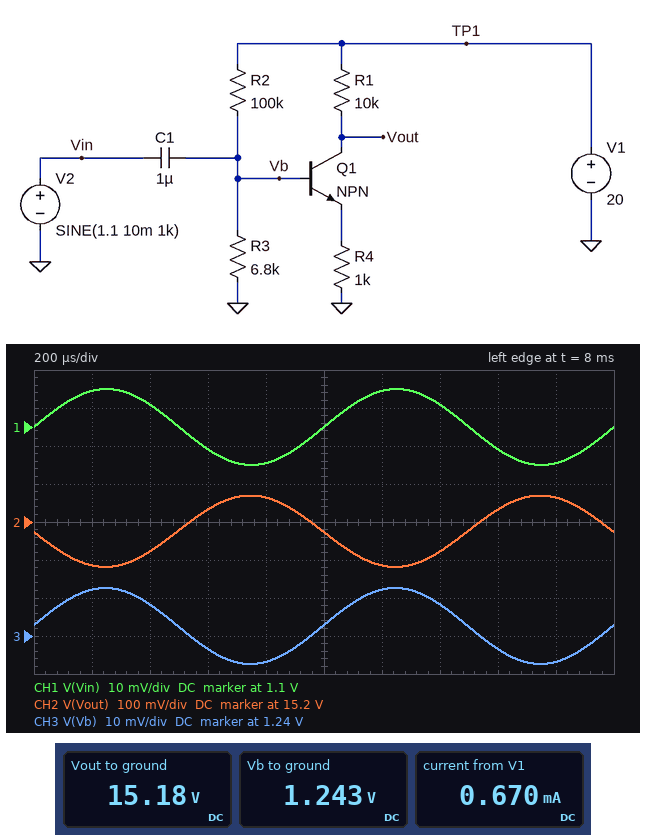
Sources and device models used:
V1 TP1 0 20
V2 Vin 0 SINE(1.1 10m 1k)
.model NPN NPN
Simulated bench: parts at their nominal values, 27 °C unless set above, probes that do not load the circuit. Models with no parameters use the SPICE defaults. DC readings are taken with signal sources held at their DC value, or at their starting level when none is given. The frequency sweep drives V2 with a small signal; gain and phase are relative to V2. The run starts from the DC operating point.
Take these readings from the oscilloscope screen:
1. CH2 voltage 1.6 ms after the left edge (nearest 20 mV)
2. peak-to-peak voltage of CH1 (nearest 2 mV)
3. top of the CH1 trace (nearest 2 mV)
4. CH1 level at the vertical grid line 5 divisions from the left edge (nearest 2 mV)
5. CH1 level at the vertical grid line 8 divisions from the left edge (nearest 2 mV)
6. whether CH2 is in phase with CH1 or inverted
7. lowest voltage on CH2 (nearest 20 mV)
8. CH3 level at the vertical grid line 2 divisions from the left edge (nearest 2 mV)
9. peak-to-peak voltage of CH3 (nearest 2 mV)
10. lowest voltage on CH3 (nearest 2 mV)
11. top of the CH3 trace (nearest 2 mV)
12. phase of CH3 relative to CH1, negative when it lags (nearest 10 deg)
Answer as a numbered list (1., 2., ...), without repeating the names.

1. 15.24 V
2. 20 mV
3. 1.110 V
4. 1.100 V
5. 1.094 V
6. inverted
7. 15.08 V
8. 1.248 V
9. 20 mV
10. 1.232 V
11. 1.252 V
12. 0 deg
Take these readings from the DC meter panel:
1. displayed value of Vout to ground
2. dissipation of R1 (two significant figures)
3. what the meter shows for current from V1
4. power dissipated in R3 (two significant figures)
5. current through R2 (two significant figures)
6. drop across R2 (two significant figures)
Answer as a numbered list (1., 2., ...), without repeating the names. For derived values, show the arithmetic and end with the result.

1. 15.18 V
2. (20 V - 15.18 V)^2 / 10 kΩ = 2.3 mW
3. 0.670 mA
4. (1.243 V)^2 / 6.8 kΩ = 230 µW
5. (20 V - 1.243 V) / 100 kΩ = 190 µA
6. 20 V - 1.243 V = 19 V
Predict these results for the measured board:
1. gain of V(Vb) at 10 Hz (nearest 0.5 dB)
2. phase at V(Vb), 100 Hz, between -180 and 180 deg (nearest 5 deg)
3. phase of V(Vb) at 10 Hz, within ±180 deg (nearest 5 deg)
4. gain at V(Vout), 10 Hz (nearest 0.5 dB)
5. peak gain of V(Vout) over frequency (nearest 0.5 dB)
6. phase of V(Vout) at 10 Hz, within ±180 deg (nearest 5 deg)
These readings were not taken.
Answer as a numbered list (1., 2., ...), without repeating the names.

1. -9.0 dB
2. 15 deg
3. 70 deg
4. 10.5 dB
5. 19.5 dB
6. -110 deg
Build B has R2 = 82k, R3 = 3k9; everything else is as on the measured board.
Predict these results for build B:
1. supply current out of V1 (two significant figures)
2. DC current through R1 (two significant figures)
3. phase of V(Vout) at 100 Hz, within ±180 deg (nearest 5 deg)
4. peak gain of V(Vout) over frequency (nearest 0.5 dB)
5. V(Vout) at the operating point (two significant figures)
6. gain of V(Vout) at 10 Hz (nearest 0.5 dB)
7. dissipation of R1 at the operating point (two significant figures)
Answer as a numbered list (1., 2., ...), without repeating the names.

1. 400 µA
2. 170 µA
3. -155 deg
4. 18.5 dB
5. 18 V
6. 5.5 dB
7. 290 µW
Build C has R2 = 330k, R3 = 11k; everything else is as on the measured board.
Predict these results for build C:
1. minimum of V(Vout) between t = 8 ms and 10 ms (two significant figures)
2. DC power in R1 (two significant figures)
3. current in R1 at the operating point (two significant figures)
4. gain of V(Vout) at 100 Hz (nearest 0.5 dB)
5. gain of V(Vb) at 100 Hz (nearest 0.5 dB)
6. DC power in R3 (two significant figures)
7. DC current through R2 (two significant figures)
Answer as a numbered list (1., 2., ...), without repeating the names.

1. 20 V
2. 290 nW
3. 5.4 µA
4. 4.5 dB
5. 0 dB
6. 38 µW
7. 59 µA
